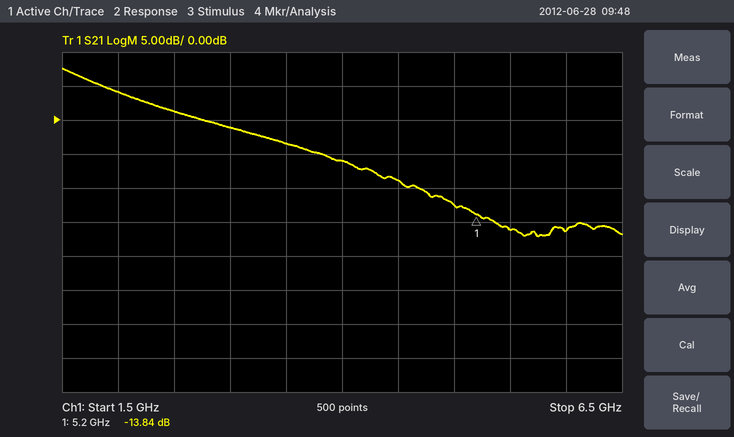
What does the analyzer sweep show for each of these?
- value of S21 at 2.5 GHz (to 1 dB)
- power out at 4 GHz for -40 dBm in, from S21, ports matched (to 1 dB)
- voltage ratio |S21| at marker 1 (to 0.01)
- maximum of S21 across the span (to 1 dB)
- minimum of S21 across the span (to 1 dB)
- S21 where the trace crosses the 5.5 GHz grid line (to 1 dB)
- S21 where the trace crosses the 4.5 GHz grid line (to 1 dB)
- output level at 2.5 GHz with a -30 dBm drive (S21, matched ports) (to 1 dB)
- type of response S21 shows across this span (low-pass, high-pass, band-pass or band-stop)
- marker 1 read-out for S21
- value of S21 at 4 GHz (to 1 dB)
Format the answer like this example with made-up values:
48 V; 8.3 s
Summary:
1 dB; -46 dBm; 0.20; 8 dB; -17 dB; -16 dB; -9 dB; -29 dBm; low-pass; -13.84 dB; -6 dB
